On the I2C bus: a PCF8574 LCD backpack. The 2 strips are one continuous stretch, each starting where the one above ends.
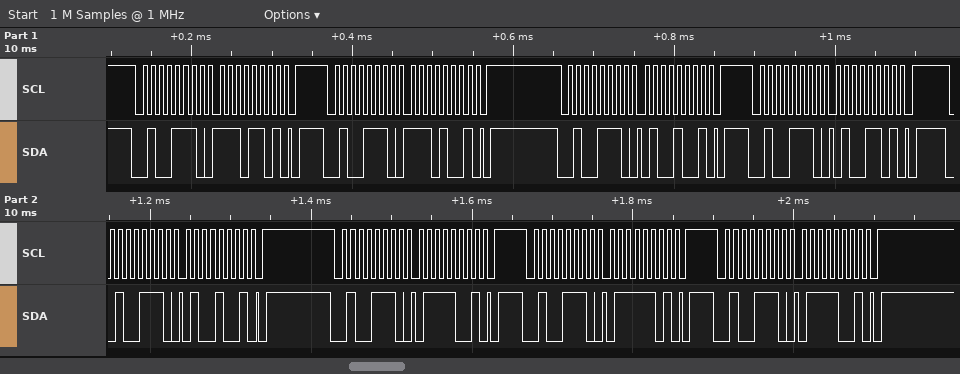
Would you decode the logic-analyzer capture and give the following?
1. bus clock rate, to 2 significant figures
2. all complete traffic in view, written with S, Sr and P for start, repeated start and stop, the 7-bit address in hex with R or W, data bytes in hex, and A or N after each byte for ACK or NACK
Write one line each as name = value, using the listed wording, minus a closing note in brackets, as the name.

bus clock rate, to 2 significant figures = 100 kHz
all complete traffic in view, written with S, Sr and P for start, repeated start and stop, the 7-bit address in hex with R or W, data bytes in hex, and A or N after each byte for ACK or NACK = S 27W A ED A P S 27W A E9 A P S 27W A 49 A P S 27W A 4D A P S 27W A 49 A P S 27W A 79 A P S 27W A 7D A P S 27W A 79 A P
